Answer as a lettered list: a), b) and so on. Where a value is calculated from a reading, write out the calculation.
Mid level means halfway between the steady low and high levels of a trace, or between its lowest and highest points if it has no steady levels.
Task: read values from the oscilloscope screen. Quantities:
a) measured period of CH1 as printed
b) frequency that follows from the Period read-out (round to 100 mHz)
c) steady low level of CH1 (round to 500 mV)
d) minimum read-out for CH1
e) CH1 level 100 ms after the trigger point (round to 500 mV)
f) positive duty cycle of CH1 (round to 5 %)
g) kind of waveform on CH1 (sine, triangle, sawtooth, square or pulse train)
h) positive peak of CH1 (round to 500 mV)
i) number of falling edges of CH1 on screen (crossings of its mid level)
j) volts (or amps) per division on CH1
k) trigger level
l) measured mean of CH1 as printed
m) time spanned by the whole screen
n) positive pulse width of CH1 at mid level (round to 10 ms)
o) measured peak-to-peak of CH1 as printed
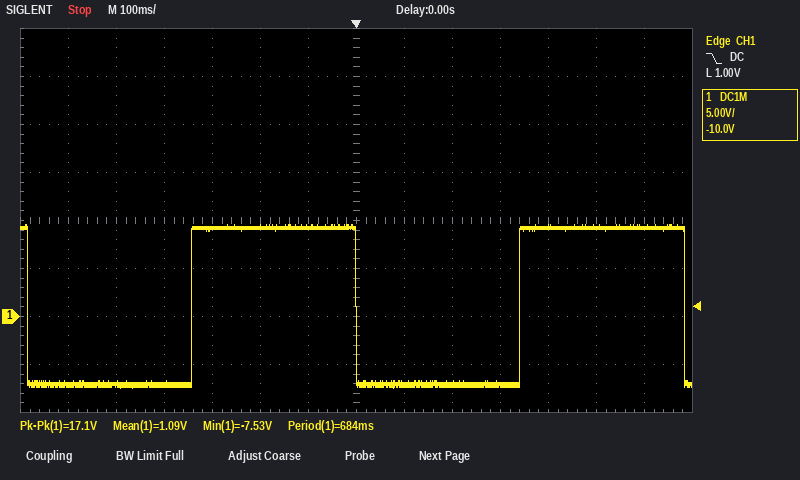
a) 684 ms
b) 1 / 684 ms ≈ 1.5 Hz
c) -7.0 V
d) -7.53 V
e) -7.0 V
f) 50 %
g) square
h) 9.5 V
i) 3
j) 5 V
k) 1.00 V
l) 1.09 V
m) 1.4 s
n) 340 ms
o) 17.1 V
